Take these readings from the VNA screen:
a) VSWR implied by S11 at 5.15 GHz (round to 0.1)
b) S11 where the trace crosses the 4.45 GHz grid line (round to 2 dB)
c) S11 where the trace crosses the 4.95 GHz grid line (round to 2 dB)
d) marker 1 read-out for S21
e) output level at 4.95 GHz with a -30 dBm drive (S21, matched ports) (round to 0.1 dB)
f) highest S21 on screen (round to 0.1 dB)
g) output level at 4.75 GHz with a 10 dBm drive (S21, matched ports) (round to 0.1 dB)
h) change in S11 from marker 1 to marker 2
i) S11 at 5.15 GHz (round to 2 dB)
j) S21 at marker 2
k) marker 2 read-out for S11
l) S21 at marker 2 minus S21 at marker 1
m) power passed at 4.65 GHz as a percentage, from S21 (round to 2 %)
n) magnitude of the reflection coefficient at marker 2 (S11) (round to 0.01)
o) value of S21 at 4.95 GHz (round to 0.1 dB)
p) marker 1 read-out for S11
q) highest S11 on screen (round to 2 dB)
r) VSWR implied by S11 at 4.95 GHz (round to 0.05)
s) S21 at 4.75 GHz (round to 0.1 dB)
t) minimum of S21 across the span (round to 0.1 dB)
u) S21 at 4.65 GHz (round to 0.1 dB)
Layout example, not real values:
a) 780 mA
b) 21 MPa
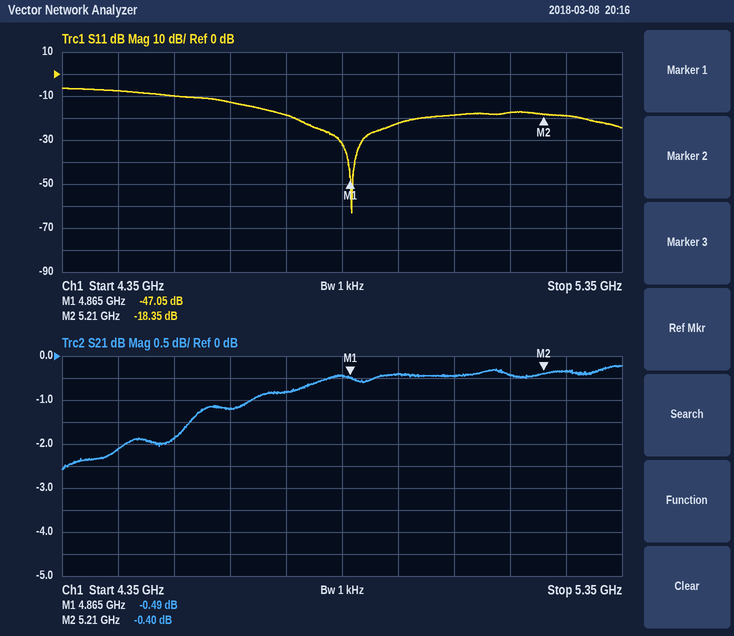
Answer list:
a) 1.3
b) -8 dB
c) -22 dB
d) -0.49 dB
e) -30.4 dBm
f) -0.2 dB
g) 9.2 dBm
h) 28.70 dB
i) -18 dB
j) -0.40 dB
k) -18.35 dB
l) 0.09 dB
m) 76 %
n) 0.12
o) -0.4 dB
p) -47.05 dB
q) -6 dB
r) 1.15
s) -0.8 dB
t) -2.6 dB
u) -1.2 dB
